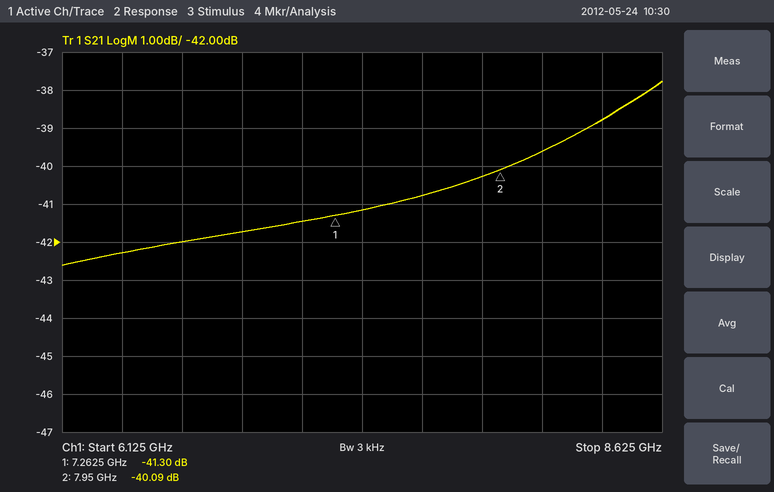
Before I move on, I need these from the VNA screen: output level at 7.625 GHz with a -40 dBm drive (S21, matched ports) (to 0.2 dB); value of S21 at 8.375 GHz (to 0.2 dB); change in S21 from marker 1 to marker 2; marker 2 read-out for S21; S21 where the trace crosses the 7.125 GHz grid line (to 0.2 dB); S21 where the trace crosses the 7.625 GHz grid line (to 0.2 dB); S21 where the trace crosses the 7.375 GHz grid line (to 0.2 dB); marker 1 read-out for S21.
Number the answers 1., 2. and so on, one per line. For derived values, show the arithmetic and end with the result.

1. -40 dBm + (-40.8 dB) = -80.8 dBm
2. -38.8 dB
3. -40.09 − (-41.3) = 1.21 dB
4. -40.09 dB
5. -41.4 dB
6. -40.8 dB
7. -41.2 dB
8. -41.30 dB
